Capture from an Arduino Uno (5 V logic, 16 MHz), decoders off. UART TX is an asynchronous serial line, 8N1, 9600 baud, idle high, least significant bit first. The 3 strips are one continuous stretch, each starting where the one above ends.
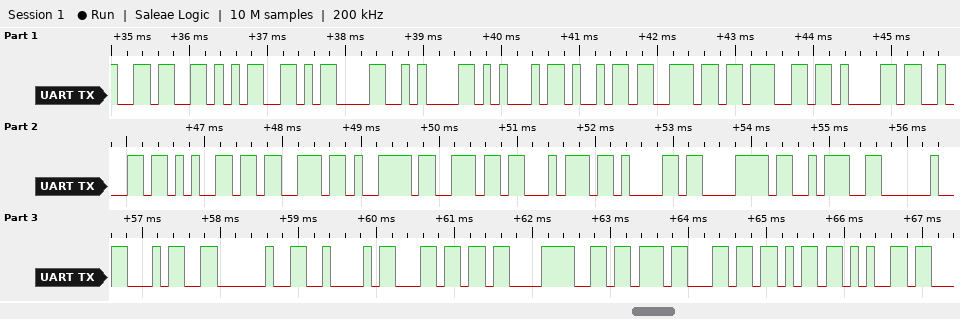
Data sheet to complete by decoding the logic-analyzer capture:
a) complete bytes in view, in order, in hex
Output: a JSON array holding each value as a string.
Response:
["36 35 0D 0A 45 69 6E 67 61 62 65 73 79 6E 74 61 78 3A 20 34 20 42 6C C3 B6 63 6B 65"]
